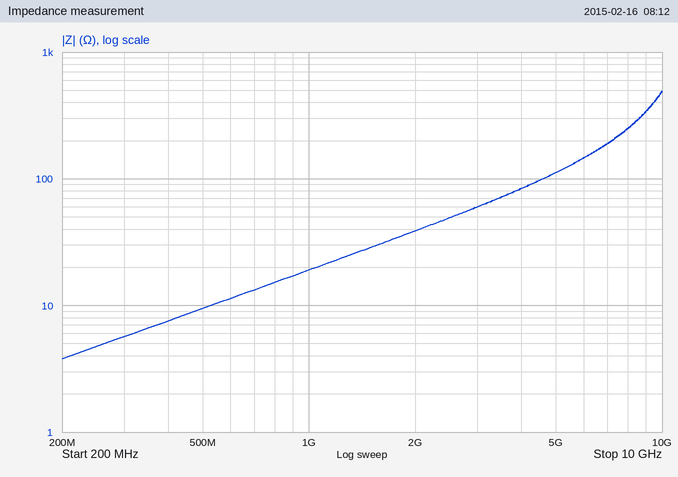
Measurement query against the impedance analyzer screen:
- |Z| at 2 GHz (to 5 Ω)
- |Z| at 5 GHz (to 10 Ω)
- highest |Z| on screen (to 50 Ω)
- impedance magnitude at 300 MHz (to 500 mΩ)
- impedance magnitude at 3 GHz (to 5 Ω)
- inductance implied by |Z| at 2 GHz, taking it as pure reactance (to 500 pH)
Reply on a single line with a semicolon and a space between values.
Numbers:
40 Ω; 110 Ω; 500 Ω; 5.5 Ω; 60 Ω; 3.0 nH
